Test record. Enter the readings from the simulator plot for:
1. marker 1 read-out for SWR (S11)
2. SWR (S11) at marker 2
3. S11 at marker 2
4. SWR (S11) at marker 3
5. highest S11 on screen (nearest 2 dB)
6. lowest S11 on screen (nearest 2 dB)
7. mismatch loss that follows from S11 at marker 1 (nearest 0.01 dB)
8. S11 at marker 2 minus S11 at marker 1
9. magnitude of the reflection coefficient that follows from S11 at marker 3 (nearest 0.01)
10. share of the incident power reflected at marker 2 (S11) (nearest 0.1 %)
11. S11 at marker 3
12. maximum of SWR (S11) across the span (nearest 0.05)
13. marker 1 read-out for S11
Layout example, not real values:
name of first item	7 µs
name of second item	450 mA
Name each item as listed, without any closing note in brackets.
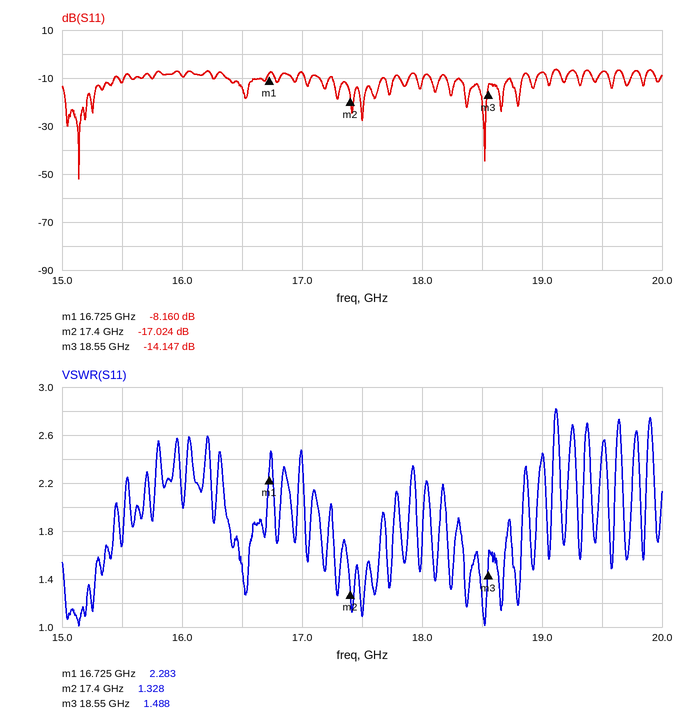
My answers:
marker 1 read-out for SWR	2.283
SWR (S11) at marker 2	1.328
S11 at marker 2	-17.024 dB
SWR (S11) at marker 3	1.488
highest S11 on screen	-6 dB
lowest S11 on screen	-52 dB
mismatch loss that follows from S11 at marker 1	0.72 dB
S11 at marker 2 minus S11 at marker 1	-8.864 dB
magnitude of the reflection coefficient that follows from S11 at marker 3	0.20
share of the incident power reflected at marker 2 (S11)	2.0 %
S11 at marker 3	-14.147 dB
maximum of SWR (S11) across the span	2.80
marker 1 read-out for S11	-8.160 dB
